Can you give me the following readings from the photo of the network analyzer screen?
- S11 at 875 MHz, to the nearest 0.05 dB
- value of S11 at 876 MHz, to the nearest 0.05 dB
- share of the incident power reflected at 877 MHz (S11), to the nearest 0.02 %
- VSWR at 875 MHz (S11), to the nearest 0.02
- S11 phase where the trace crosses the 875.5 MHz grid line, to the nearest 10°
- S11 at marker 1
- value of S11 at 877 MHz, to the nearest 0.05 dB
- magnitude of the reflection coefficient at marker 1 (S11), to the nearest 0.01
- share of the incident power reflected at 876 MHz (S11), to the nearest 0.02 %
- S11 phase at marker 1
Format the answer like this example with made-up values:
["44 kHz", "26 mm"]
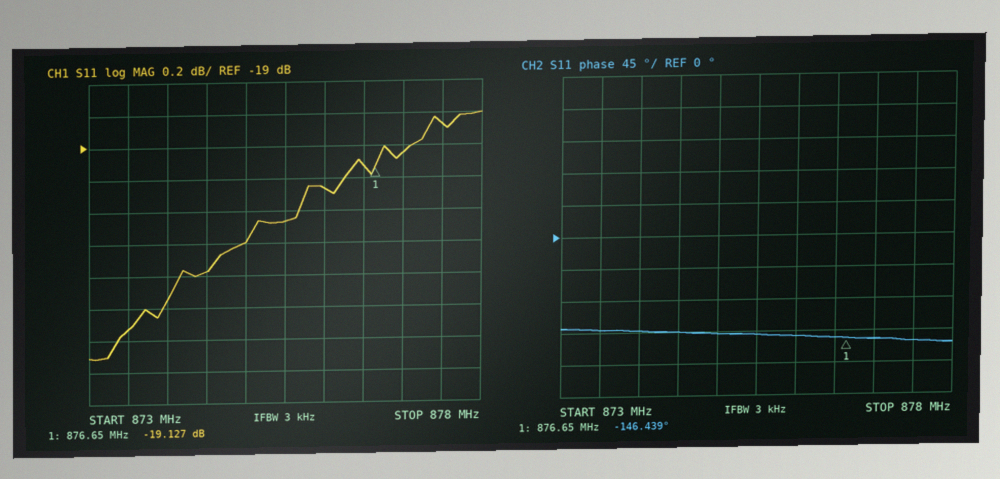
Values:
["-19.60 dB", "-19.25 dB", "1.24 %", "1.24", "-140°", "-19.127 dB", "-19.05 dB", "0.11", "1.18 %", "-146.439°"]
